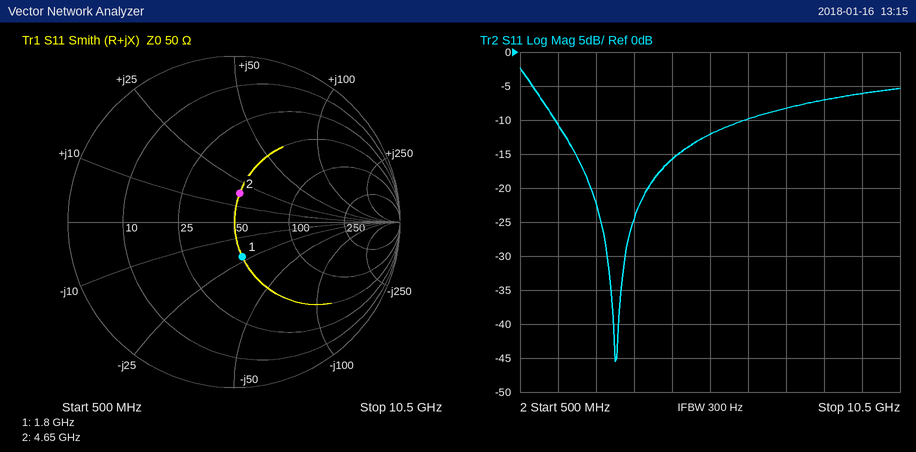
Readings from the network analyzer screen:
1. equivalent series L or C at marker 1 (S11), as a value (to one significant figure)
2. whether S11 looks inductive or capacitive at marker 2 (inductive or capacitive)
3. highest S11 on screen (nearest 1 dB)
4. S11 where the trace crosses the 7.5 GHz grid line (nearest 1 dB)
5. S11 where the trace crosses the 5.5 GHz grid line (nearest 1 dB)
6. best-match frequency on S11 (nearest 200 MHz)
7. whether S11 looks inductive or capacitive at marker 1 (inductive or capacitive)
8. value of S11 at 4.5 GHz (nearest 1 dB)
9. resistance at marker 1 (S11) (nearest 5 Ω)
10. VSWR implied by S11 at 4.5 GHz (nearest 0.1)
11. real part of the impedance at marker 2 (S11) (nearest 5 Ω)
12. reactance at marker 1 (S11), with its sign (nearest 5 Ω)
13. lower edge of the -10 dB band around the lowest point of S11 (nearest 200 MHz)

4 pF
inductive
-2 dB
-8 dB
-12 dB
3.0 GHz
capacitive
-16 dB
50 Ω
1.4
50 Ω
-20 Ω
1.4 GHz
